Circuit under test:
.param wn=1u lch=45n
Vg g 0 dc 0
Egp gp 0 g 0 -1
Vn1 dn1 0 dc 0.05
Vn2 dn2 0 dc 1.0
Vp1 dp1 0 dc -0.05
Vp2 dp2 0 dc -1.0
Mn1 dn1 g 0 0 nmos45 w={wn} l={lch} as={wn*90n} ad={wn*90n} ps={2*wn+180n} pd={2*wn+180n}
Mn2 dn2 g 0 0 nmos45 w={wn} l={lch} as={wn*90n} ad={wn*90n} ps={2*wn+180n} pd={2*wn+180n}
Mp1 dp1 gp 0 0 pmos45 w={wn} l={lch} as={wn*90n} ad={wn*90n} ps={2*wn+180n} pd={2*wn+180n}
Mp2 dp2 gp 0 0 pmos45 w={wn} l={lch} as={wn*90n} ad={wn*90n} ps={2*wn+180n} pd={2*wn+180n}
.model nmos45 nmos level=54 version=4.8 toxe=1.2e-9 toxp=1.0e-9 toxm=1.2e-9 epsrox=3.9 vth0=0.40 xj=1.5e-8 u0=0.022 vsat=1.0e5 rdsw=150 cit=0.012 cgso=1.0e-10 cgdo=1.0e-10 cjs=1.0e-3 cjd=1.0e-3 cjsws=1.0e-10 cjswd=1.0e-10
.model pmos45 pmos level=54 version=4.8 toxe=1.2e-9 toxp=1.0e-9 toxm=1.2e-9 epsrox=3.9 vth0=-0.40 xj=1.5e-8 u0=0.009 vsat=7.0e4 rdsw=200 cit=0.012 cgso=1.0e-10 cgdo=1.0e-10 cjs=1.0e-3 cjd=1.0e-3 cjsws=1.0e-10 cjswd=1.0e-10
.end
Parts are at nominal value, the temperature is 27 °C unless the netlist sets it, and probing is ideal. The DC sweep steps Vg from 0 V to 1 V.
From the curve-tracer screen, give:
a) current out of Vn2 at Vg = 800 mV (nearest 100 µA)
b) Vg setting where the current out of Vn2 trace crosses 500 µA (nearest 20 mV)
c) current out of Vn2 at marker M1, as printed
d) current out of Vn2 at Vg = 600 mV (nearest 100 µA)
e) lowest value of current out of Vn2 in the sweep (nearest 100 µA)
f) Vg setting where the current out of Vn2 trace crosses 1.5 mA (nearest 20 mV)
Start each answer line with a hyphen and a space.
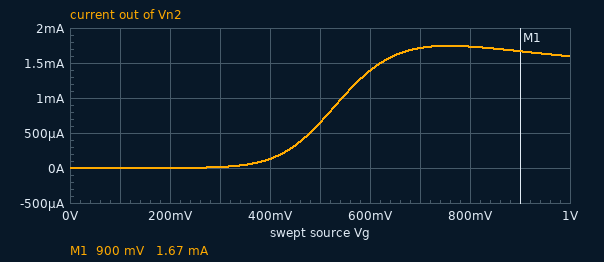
- 1.7 mA
- 480 mV
- 1.67 mA
- 1.4 mA
- 0 A
- 620 mV
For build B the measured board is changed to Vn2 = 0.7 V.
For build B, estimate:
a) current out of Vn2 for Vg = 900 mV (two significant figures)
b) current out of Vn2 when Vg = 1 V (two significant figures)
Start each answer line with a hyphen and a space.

- 670 µA
- 810 µA
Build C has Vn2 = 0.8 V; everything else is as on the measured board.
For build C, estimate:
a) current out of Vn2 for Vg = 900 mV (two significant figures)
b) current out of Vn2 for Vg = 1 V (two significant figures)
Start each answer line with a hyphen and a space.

- 770 µA
- 890 µA
